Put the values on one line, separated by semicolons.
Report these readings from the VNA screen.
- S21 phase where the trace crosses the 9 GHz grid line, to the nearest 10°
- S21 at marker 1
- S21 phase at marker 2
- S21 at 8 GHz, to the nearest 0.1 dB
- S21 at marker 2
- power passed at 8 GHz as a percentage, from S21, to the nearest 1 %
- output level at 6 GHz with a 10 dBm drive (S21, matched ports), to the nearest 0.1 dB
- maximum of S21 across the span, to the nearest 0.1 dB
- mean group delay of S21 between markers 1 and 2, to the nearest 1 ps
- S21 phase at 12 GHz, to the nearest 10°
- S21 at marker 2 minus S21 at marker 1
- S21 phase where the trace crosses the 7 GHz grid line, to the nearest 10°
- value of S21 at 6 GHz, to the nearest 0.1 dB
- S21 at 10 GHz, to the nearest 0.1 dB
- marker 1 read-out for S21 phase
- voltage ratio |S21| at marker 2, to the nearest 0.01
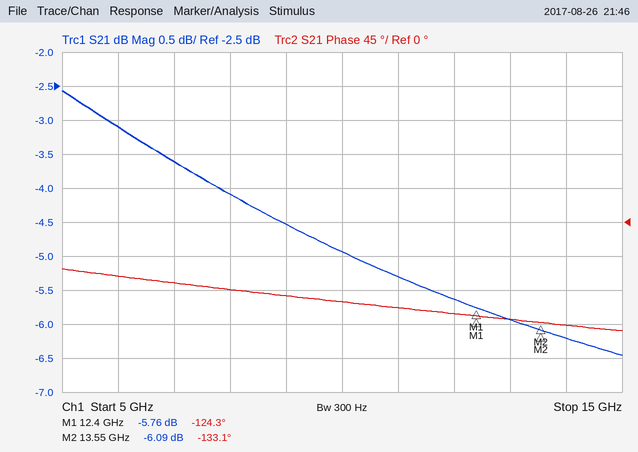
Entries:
-100°; -5.76 dB; -133.1°; -4.1 dB; -6.09 dB; 39 %; 6.9 dBm; -2.6 dB; 21 ps; -120°; -0.33 dB; -80°; -3.1 dB; -4.9 dB; -124.3°; 0.50
